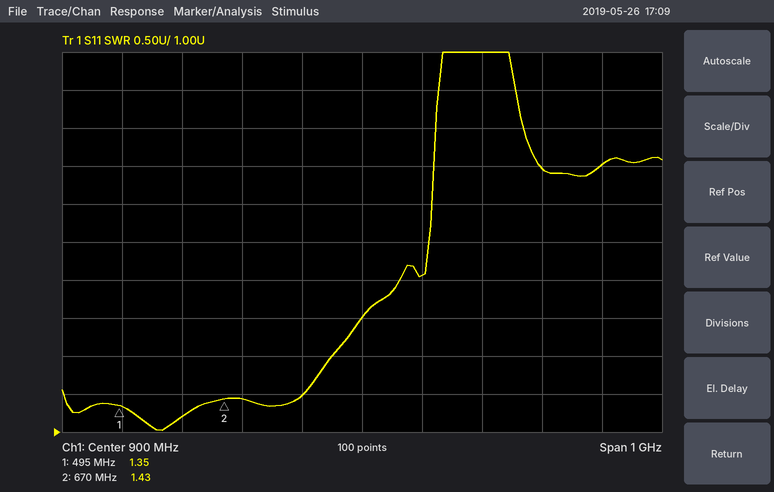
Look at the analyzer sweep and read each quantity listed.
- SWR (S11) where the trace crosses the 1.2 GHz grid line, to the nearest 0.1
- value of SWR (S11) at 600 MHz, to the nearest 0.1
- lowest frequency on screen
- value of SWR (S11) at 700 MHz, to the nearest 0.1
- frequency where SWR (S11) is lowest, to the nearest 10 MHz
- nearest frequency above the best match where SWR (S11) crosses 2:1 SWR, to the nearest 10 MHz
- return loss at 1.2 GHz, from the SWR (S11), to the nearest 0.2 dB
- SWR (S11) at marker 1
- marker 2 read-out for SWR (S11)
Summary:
4.5
1.2
400 MHz
1.4
570 MHz
850 MHz
4.0 dB
1.35
1.43
